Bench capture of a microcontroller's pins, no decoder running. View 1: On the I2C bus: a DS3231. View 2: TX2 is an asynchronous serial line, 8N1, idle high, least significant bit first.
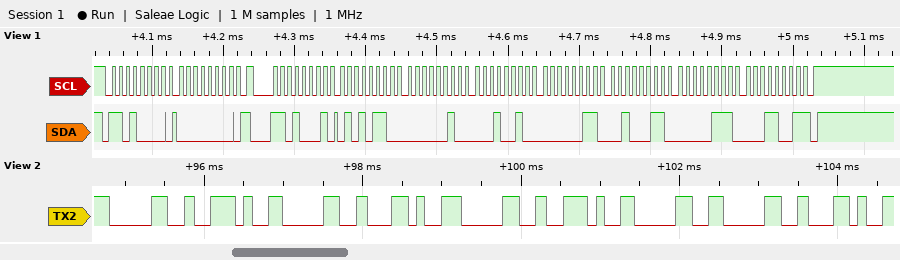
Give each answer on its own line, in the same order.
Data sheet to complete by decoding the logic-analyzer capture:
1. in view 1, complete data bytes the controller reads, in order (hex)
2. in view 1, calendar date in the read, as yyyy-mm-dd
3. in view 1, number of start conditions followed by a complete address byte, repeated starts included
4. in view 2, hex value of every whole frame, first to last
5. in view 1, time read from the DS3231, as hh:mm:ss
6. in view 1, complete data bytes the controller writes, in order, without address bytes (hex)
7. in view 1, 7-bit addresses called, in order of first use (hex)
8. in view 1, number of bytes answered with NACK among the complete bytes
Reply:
56 02 12 03 23 07 19
2019-07-23
2
30 2E 30 2C 30 2E 30 30 2C
12:02:56
00
0x68
1
